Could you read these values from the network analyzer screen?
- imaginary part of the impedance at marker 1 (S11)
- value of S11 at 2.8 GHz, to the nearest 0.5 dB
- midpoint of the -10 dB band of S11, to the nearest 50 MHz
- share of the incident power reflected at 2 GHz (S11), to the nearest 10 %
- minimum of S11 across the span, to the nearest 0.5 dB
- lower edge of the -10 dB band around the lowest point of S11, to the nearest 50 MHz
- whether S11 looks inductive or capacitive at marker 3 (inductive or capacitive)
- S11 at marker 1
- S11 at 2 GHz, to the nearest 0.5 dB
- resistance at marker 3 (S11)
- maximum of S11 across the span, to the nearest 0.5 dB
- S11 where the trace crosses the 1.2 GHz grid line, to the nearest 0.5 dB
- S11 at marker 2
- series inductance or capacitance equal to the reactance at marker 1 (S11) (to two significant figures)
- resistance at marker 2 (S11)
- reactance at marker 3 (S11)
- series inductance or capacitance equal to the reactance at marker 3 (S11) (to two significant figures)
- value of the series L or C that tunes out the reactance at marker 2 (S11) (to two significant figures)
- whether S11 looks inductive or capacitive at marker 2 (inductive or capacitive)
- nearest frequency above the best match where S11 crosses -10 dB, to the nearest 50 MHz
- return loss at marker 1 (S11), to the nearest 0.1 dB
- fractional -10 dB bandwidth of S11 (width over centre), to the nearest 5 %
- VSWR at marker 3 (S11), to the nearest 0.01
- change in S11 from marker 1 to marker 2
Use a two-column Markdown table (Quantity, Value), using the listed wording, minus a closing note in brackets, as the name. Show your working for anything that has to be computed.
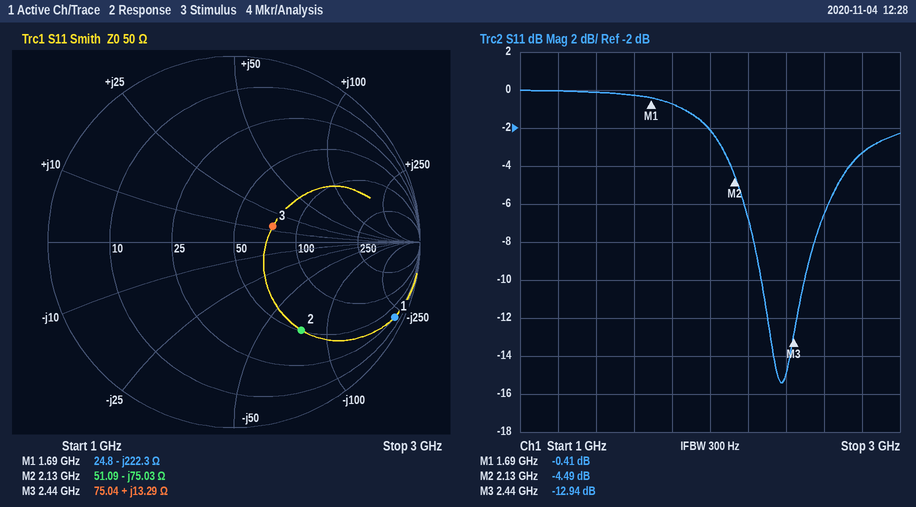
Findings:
| Quantity | Value |
|---|---|
| imaginary part of the impedance at marker 1 | -222.3 Ω |
| value of S11 at 2.8 GHz, to the nearest 0.5 dB | -3.5 dB |
| midpoint of the -10 dB band of S11, to the nearest 50 MHz | 2.40 GHz |
| share of the incident power reflected at 2 GHz (S11), to the nearest 10 % | 10^(-2/10) ≈ 63.1 %, so 60 % to the nearest 10 % |
| minimum of S11 across the span, to the nearest 0.5 dB | -15.5 dB |
| lower edge of the -10 dB band around the lowest point of S11, to the nearest 50 MHz | 2.25 GHz |
| whether S11 looks inductive or capacitive at marker 3 | inductive |
| S11 at marker 1 | -0.41 dB |
| S11 at 2 GHz, to the nearest 0.5 dB | -2.0 dB |
| resistance at marker 3 | 75.04 Ω |
| maximum of S11 across the span, to the nearest 0.5 dB | 0.0 dB |
| S11 where the trace crosses the 1.2 GHz grid line, to the nearest 0.5 dB | 0.0 dB |
| S11 at marker 2 | -4.49 dB |
| series inductance or capacitance equal to the reactance at marker 1 (S11) | C = 1/(2π × 1.69 GHz × 222.3 Ω) ≈ 424 fF, so 420 fF to two significant figures |
| resistance at marker 2 | 51.09 Ω |
| reactance at marker 3 | +13.29 Ω |
| series inductance or capacitance equal to the reactance at marker 3 (S11) | L = 13.29 Ω/(2π × 2.44 GHz) ≈ 867 pH, so 870 pH to two significant figures |
| value of the series L or C that tunes out the reactance at marker 2 (S11) | L = 75.03 Ω/(2π × 2.13 GHz) ≈ 5.6 nH |
| whether S11 looks inductive or capacitive at marker 2 | capacitive |
| nearest frequency above the best match where S11 crosses -10 dB, to the nearest 50 MHz | 2.50 GHz |
| return loss at marker 1 (S11), to the nearest 0.1 dB | 0.4 dB |
| fractional -10 dB bandwidth of S11 (width over centre), to the nearest 5 % | 250 MHz / 2.375 GHz ≈ 10 % |
| VSWR at marker 3 (S11), to the nearest 0.01 | 1.58 |
| change in S11 from marker 1 to marker 2 | -4.49 − (-0.41) = -4.08 dB |
